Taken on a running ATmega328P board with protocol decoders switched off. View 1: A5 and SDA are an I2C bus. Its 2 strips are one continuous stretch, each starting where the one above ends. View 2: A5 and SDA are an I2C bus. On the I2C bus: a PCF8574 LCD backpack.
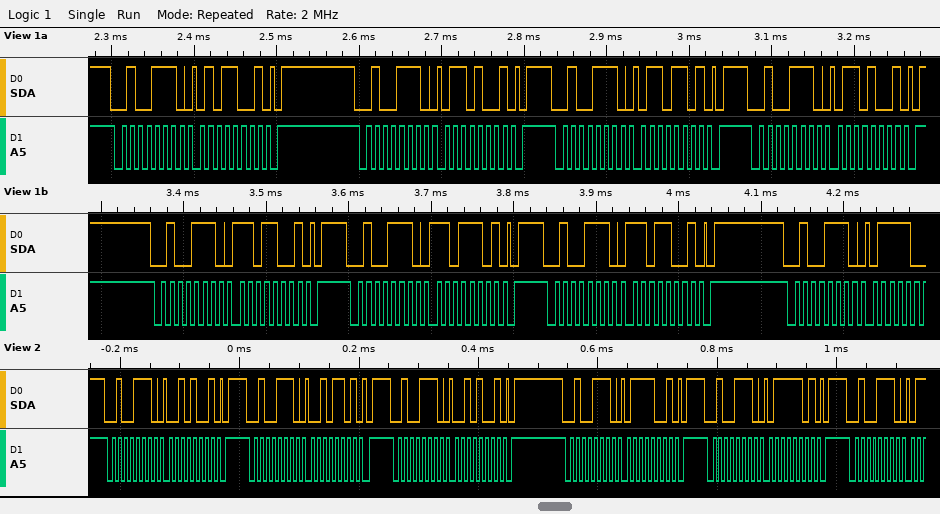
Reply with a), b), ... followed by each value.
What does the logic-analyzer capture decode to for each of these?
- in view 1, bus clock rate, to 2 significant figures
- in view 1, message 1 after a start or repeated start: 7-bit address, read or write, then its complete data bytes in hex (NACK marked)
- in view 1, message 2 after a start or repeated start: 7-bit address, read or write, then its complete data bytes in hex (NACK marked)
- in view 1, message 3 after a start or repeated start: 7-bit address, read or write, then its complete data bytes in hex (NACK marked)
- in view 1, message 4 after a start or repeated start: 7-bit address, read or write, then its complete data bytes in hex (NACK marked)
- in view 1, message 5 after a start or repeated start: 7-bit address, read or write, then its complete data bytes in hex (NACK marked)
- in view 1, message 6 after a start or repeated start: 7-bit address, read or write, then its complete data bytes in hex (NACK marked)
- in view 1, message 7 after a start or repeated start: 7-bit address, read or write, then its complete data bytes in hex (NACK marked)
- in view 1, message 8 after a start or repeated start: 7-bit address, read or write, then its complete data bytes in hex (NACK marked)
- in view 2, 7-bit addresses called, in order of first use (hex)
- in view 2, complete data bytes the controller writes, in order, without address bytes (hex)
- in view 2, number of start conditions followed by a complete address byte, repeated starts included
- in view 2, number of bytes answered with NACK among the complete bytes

a) 100 kHz
b) 0x27 write: 59
c) 0x27 write: 69
d) 0x27 write: 6D
e) 0x27 write: 69
f) 0x27 write: D9
g) 0x27 write: DD
h) 0x27 write: D9
i) 0x27 write
j) 0x27
k) 29 2D 29 79 7D
l) 6
m) 0
